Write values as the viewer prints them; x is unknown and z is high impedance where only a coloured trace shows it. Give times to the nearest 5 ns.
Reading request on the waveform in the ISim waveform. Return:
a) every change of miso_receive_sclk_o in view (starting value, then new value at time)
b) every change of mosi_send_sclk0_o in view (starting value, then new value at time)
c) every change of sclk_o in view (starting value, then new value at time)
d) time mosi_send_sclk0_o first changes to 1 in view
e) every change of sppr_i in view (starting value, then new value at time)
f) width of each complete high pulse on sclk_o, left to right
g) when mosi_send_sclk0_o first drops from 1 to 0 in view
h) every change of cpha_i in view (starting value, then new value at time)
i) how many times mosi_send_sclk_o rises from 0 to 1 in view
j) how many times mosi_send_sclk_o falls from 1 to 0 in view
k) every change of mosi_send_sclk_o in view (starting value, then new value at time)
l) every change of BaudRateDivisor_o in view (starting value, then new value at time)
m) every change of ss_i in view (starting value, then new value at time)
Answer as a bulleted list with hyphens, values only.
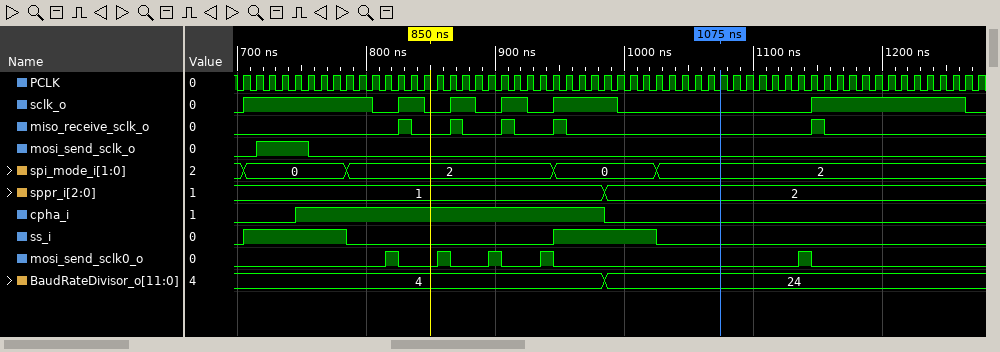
- 0, 1 at 825 ns, 0 at 835 ns, 1 at 865 ns, 0 at 875 ns, 1 at 905 ns, 0 at 915 ns, 1 at 945 ns, 0 at 955 ns, 1 at 1145 ns, 0 at 1155 ns
- 0, 1 at 815 ns, 0 at 825 ns, 1 at 855 ns, 0 at 865 ns, 1 at 895 ns, 0 at 905 ns, 1 at 935 ns, 0 at 945 ns, 1 at 1135 ns, 0 at 1145 ns
- 0, 1 at 705 ns, 0 at 805 ns, 1 at 825 ns, 0 at 845 ns, 1 at 865 ns, 0 at 885 ns, 1 at 905 ns, 0 at 925 ns, 1 at 945 ns, 0 at 995 ns, 1 at 1145 ns, 0 at 1265 ns
- 815 ns
- 1, 2 at 985 ns
- 100 ns, 20 ns, 20 ns, 20 ns, 50 ns, 120 ns
- 825 ns
- 0, 1 at 745 ns, 0 at 985 ns
- 1
- 1
- 0, 1 at 715 ns, 0 at 755 ns
- 4, 24 at 985 ns
- 0, 1 at 705 ns, 0 at 785 ns, 1 at 945 ns, 0 at 1025 ns
